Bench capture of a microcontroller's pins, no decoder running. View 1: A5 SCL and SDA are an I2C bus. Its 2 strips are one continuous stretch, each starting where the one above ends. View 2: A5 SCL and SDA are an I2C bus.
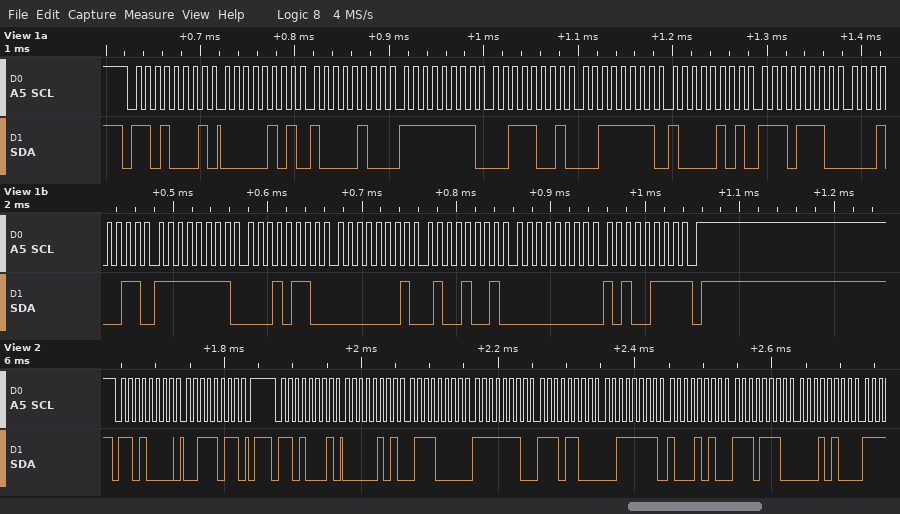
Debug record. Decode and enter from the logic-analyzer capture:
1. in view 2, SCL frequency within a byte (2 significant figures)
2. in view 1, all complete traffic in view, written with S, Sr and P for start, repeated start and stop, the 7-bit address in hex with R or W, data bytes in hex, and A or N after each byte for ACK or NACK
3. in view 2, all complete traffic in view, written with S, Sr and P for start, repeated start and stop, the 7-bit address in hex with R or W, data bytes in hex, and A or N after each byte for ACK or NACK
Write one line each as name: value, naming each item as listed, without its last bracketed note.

in view 2, SCL frequency within a byte: 100 kHz
in view 1, all complete traffic in view, written with S, Sr and P for start, repeated start and stop, the 7-bit address in hex with R or W, data bytes in hex, and A or N after each byte for ACK or NACK: S 68R A 05 A 84 A FF A 39 A 3F A 85 A EE A 13 A FF A 16 A 01 A 49 A 00 A A7 N P
in view 2, all complete traffic in view, written with S, Sr and P for start, repeated start and stop, the 7-bit address in hex with R or W, data bytes in hex, and A or N after each byte for ACK or NACK: S 68W A 3B A P S 68R A 05 A 70 A FE A EC A 3F A 8A A EE A 14 A
